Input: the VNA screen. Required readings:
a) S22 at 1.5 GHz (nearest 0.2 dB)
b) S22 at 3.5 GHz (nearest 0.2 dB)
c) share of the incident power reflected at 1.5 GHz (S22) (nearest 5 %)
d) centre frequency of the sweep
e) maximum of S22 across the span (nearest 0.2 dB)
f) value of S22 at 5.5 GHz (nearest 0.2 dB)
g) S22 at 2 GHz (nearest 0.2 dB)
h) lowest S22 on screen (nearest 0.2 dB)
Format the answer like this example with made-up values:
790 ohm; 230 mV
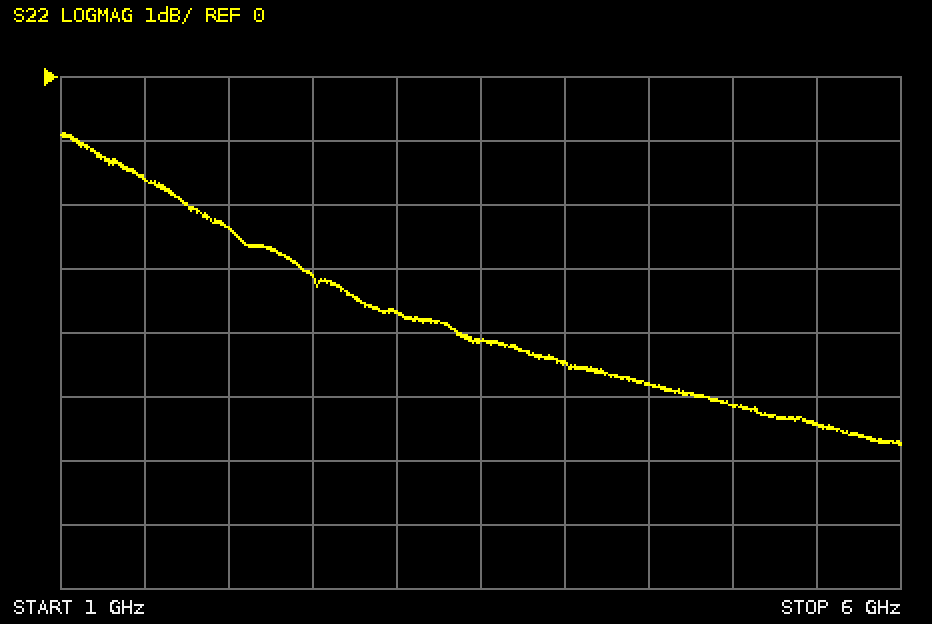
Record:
-1.6 dB; -4.2 dB; 70 %; 3.5 GHz; -0.8 dB; -5.4 dB; -2.4 dB; -5.8 dB
